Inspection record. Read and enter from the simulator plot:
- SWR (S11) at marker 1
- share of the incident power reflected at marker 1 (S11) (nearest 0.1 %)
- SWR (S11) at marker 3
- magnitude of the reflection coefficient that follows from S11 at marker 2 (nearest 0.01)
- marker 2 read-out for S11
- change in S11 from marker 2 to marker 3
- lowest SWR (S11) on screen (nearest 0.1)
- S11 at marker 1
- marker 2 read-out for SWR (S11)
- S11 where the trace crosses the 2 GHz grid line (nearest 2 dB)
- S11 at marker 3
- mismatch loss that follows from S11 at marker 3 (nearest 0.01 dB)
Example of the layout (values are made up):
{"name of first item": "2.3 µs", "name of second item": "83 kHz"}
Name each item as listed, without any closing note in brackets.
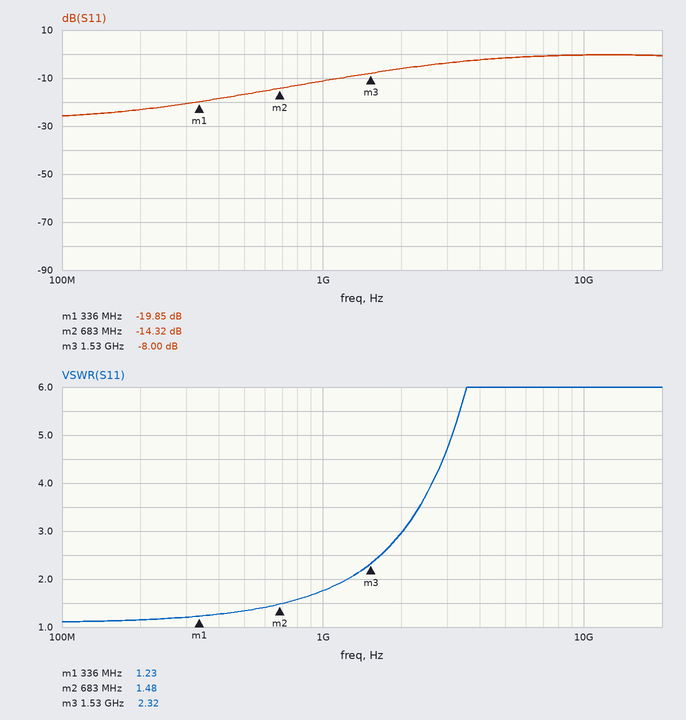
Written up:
{"SWR (S11) at marker 1": "1.23", "share of the incident power reflected at marker 1 (S11)": "1.0 %", "SWR (S11) at marker 3": "2.32", "magnitude of the reflection coefficient that follows from S11 at marker 2": "0.19", "marker 2 read-out for S11": "-14.32 dB", "change in S11 from marker 2 to marker 3": "6.32 dB", "lowest SWR (S11) on screen": "1.1", "S11 at marker 1": "-19.85 dB", "marker 2 read-out for SWR": "1.48", "S11 where the trace crosses the 2 GHz grid line": "-6 dB", "S11 at marker 3": "-8.00 dB", "mismatch loss that follows from S11 at marker 3": "0.75 dB"}
